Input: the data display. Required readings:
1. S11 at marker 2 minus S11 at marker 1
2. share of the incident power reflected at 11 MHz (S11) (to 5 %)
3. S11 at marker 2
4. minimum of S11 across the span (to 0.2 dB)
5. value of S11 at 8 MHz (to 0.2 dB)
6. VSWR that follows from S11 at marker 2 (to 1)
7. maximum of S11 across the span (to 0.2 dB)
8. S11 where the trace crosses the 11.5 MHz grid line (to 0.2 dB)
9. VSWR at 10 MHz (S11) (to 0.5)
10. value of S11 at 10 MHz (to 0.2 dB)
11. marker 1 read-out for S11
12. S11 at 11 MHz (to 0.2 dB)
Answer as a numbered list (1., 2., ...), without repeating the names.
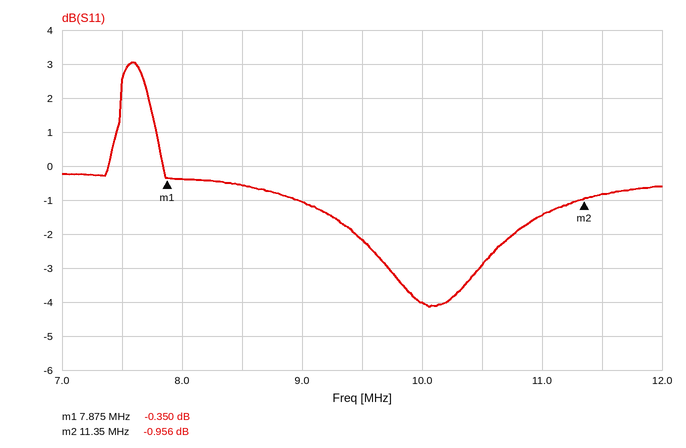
1. -0.606 dB
2. 70 %
3. -0.956 dB
4. -4.2 dB
5. -0.4 dB
6. 18
7. 3.0 dB
8. -0.8 dB
9. 4.5
10. -4.0 dB
11. -0.350 dB
12. -1.4 dB
